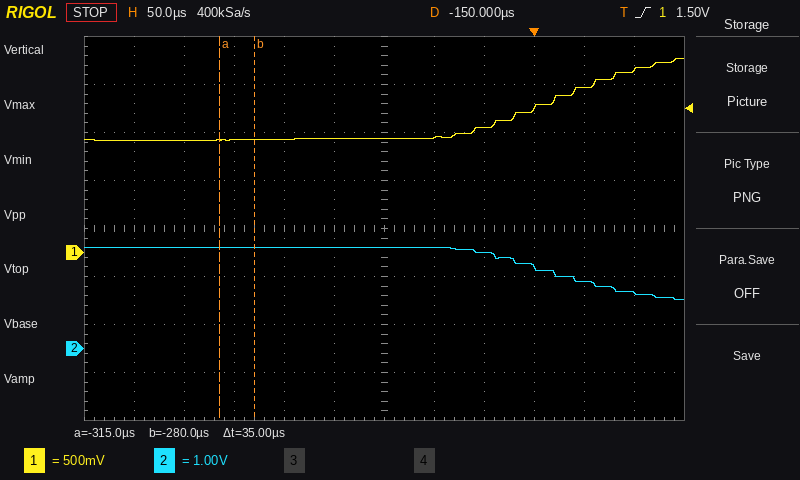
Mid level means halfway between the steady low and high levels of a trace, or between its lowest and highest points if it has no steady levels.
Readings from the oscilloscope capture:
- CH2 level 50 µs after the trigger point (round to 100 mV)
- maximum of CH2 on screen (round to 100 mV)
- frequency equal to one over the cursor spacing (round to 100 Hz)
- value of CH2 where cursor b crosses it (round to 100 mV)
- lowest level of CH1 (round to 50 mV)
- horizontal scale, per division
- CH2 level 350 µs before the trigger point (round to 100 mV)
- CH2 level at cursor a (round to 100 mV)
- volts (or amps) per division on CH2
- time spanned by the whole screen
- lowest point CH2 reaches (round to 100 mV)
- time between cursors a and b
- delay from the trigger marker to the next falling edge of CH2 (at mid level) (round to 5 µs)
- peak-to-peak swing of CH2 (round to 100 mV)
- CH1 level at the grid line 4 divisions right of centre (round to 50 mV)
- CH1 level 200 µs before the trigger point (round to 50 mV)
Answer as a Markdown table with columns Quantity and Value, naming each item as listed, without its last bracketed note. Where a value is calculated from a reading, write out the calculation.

| Quantity | Value |
|---|---|
| CH2 level 50 µs after the trigger point | 1.4 V |
| maximum of CH2 on screen | 2.1 V |
| frequency equal to one over the cursor spacing | 1 / 35 µs ≈ 28.6 kHz |
| value of CH2 where cursor b crosses it | 2.1 V |
| lowest level of CH1 | 1.15 V |
| horizontal scale, per division | 50 µs |
| CH2 level 350 µs before the trigger point | 2.1 V |
| CH2 level at cursor a | 2.1 V |
| volts (or amps) per division on CH2 | 1 V |
| time spanned by the whole screen | 600 µs |
| lowest point CH2 reaches | 1.0 V |
| time between cursors a and b | 35 µs |
| delay from the trigger marker to the next falling edge of CH2 (at mid level) | 20 µs |
| peak-to-peak swing of CH2 | 2.1 V − (1.0 V) = 1.1 V |
| CH1 level at the grid line 4 divisions right of centre | 1.70 V |
| CH1 level 200 µs before the trigger point | 1.20 V |
